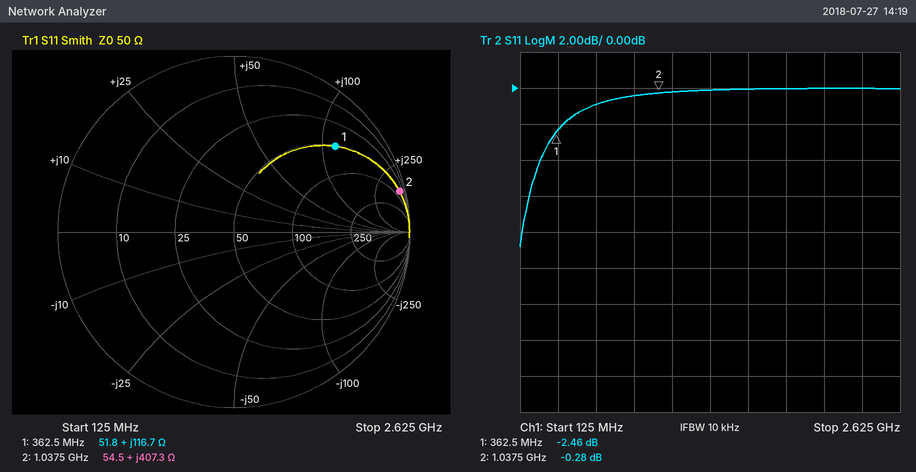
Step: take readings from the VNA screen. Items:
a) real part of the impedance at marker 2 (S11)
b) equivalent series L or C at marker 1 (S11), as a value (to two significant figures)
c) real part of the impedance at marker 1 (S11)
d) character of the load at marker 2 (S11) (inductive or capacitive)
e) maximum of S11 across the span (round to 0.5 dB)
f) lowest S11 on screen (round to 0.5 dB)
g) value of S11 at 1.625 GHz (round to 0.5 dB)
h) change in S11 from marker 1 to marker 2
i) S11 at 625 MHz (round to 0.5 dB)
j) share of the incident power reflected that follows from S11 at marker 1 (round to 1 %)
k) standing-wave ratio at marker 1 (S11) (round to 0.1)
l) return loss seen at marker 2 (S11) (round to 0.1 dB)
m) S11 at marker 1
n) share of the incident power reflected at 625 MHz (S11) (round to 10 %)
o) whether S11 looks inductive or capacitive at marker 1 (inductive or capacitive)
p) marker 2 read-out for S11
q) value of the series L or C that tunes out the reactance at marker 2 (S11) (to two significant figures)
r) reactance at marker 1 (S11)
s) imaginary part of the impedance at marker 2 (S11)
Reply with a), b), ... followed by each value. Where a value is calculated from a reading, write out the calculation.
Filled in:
a) 54.5 Ω
b) L = 116.7 Ω/(2π × 362.5 MHz) ≈ 51 nH
c) 51.8 Ω
d) inductive
e) 0.0 dB
f) -9.0 dB
g) 0.0 dB
h) -0.28 − (-2.46) = 2.18 dB
i) -1.0 dB
j) 10^(-2.46/10) ≈ 57 %
k) 7.1
l) 0.3 dB
m) -2.46 dB
n) 10^(-1/10) ≈ 79.4 %, so 80 % to the nearest 10 %
o) inductive
p) -0.28 dB
q) C = 1/(2π × 1.0375 GHz × 407.3 Ω) ≈ 377 fF, so 380 fF to two significant figures
r) +116.7 Ω
s) +407.3 Ω
